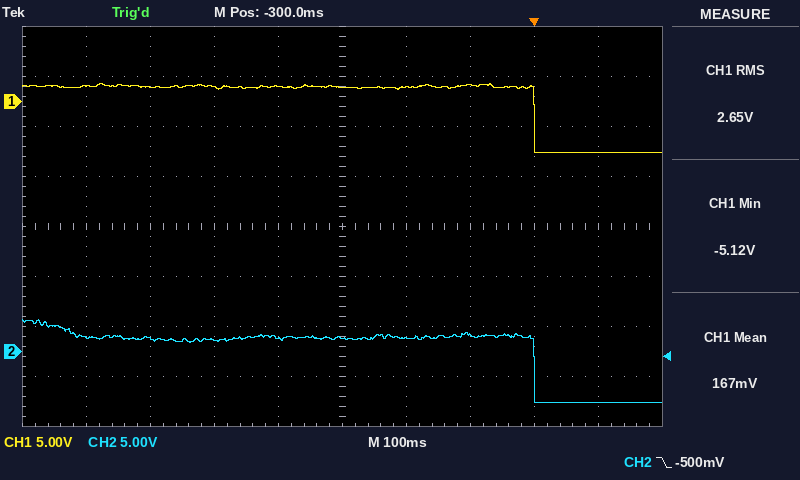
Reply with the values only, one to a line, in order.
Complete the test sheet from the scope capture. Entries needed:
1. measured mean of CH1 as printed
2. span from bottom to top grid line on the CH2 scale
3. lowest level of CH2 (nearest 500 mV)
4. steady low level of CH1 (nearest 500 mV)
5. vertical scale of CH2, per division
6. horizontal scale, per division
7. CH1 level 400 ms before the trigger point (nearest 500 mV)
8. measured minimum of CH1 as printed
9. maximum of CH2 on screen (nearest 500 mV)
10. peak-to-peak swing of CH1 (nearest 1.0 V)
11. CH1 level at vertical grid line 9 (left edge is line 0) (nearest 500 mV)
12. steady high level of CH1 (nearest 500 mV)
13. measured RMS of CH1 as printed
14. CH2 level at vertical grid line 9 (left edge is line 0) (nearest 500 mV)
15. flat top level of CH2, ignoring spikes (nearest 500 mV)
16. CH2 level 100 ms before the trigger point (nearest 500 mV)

167 mV
40 V
-5.0 V
-5.0 V
5 V
100 ms
1.5 V
-5.12 V
3.0 V
7.0 V
-5.0 V
1.5 V
2.65 V
-5.0 V
1.5 V
1.5 V
